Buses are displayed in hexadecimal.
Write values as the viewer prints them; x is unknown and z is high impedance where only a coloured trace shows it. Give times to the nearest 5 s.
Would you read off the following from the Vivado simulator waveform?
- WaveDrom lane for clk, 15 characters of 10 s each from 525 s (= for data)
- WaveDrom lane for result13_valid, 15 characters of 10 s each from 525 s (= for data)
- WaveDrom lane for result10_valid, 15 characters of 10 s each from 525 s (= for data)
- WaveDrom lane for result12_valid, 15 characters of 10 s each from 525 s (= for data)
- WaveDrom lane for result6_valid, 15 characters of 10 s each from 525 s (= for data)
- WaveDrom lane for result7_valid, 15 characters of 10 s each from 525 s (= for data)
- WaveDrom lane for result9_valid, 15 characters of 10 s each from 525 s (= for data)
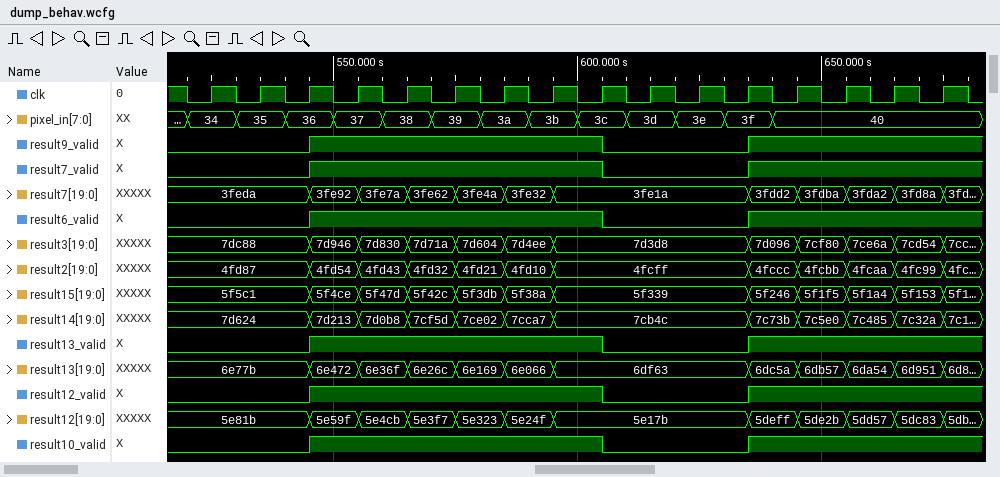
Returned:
{name: 'clk', wave: 'p..............'}
{name: 'result13_valid', wave: '0.1.....0..1...'}
{name: 'result10_valid', wave: '0.1.....0..1...'}
{name: 'result12_valid', wave: '0.1.....0..1...'}
{name: 'result6_valid', wave: '0.1.....0..1...'}
{name: 'result7_valid', wave: '0.1.....0..1...'}
{name: 'result9_valid', wave: '0.1.....0..1...'}
